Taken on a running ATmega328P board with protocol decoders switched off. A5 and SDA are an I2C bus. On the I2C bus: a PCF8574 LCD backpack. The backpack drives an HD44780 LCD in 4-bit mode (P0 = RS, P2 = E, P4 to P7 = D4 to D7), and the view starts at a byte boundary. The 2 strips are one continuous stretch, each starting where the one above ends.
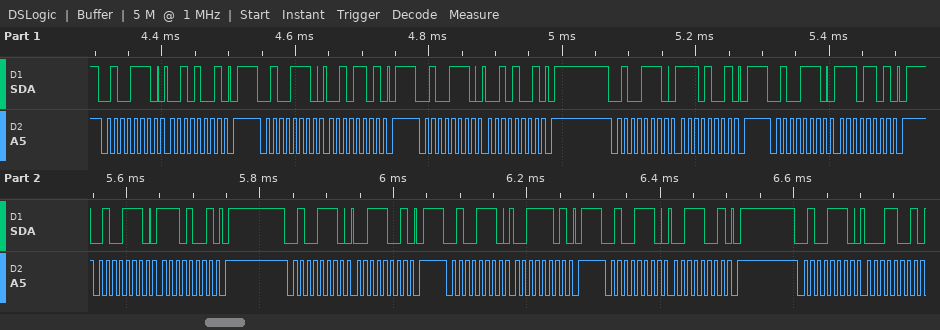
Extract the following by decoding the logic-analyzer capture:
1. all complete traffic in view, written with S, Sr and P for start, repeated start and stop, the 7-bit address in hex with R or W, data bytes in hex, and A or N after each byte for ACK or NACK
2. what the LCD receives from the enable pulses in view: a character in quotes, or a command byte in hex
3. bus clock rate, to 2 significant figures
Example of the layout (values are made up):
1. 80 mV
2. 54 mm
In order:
1. S 27W A 29 A P S 27W A 2D A P S 27W A 29 A P S 27W A E9 A P S 27W A ED A P S 27W A E9 A P S 27W A 39 A P S 27W A 3D A P S 27W A 39 A P S 27W A 19 A
2. '.'
3. 100 kHz
